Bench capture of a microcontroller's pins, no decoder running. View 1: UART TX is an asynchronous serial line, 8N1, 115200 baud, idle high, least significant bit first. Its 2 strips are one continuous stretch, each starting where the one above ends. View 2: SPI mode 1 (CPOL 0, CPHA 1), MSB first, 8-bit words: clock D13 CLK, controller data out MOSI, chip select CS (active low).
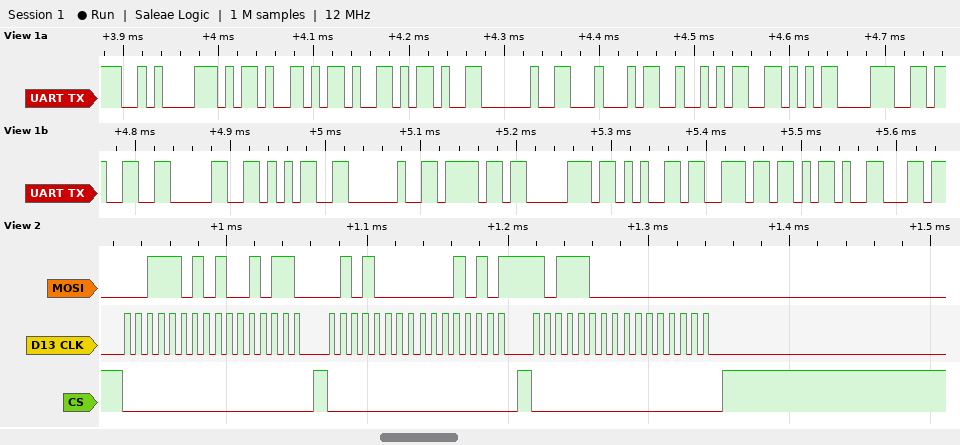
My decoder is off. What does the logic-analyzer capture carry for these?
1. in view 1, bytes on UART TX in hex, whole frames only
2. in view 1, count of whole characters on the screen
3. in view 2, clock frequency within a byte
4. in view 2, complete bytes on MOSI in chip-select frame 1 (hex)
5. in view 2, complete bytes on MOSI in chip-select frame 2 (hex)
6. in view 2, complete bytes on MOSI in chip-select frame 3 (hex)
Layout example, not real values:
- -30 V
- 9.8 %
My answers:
- 0x0A 0x2D 0x2D 0x2D 0x20 0x44 0x52 0x56 0x38 0x33 0x30 0x35 0x20 0x6F 0x70 0x65 0x6E 0x2D
- 18
- 125 kHz
- 3A 96
- 50 15
- B8 00
